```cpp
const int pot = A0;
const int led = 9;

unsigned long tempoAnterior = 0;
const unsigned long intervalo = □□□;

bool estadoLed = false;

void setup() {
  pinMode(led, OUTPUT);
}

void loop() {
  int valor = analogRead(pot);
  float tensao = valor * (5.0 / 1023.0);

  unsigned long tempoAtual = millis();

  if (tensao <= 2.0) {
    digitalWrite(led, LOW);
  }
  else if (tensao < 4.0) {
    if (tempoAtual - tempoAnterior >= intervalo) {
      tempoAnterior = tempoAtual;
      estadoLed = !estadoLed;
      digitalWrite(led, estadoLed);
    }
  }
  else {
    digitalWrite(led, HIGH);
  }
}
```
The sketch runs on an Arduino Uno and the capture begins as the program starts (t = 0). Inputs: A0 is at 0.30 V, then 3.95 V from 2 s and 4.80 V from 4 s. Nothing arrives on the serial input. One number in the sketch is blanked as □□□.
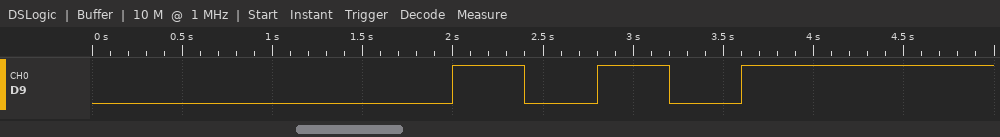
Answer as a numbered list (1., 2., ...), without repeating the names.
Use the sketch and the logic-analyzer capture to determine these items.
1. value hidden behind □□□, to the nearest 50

1. 400
